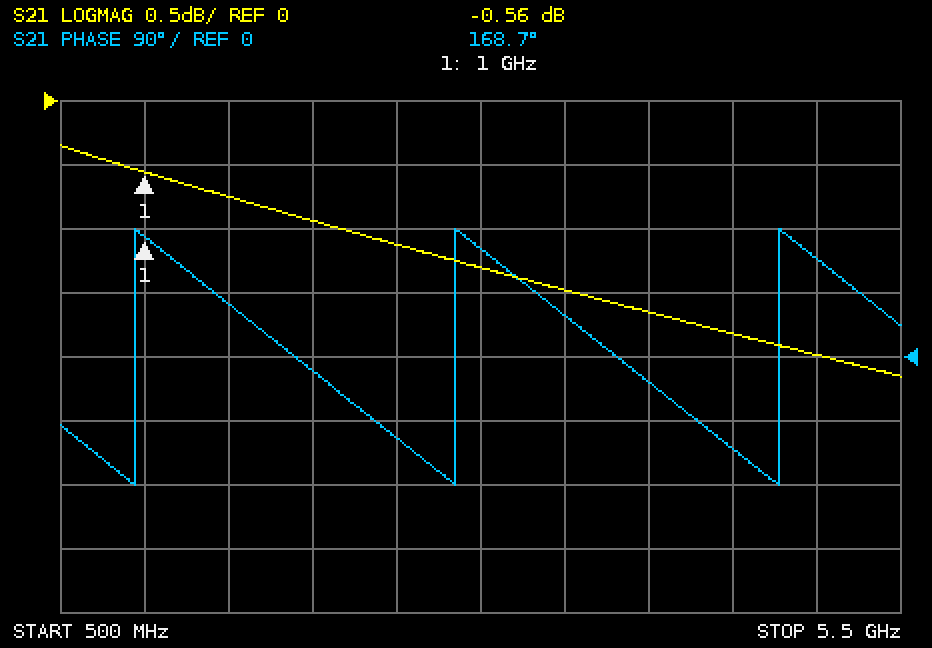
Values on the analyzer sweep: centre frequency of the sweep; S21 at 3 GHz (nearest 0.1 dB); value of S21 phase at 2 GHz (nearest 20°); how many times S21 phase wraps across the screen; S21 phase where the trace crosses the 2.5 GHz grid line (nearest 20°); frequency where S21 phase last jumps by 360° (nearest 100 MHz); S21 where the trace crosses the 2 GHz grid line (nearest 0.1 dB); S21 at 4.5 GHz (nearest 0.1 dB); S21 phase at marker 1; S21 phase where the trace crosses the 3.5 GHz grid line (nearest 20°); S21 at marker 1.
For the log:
3 GHz
-1.3 dB
-20°
3
-120°
4.8 GHz
-0.9 dB
-1.8 dB
168.7°
60°
-0.56 dB
